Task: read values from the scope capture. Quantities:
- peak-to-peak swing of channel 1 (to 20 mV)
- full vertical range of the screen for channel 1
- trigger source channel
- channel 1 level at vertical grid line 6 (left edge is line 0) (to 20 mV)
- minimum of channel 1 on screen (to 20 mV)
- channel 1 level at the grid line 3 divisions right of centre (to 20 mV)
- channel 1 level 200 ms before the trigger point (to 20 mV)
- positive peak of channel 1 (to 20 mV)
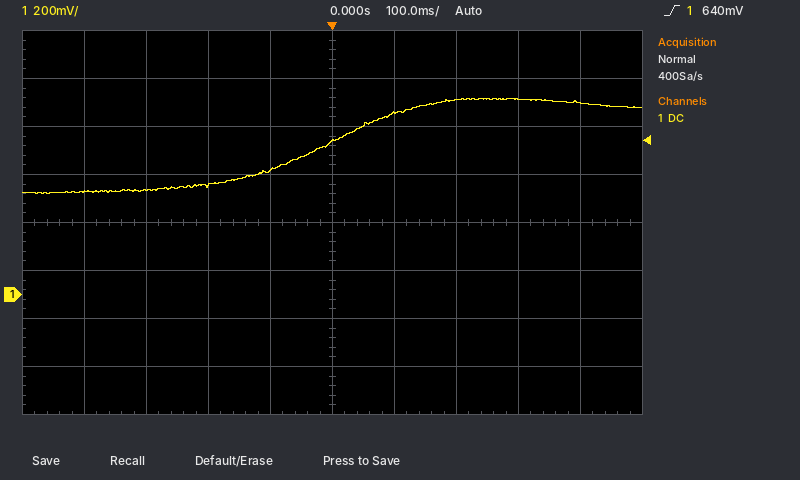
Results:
400 mV
1.6 V
channel 1
760 mV
420 mV
820 mV
460 mV
820 mV
